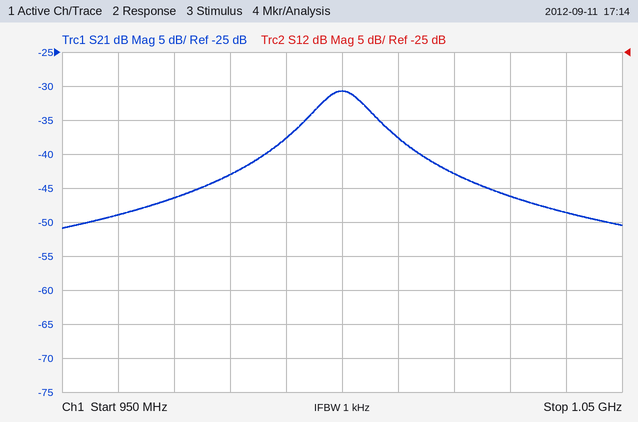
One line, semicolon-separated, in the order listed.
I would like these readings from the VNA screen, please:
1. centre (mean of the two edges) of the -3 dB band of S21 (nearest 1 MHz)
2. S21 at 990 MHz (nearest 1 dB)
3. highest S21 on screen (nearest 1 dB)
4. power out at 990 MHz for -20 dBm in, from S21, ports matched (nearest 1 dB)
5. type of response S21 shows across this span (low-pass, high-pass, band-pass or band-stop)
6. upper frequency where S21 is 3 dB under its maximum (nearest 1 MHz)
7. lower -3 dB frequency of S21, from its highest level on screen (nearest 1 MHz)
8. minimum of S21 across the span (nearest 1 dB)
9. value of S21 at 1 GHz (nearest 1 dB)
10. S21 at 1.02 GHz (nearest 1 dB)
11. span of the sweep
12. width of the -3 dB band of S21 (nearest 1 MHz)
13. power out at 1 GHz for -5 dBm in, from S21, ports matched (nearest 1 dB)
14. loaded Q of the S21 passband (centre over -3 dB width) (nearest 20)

1.000 GHz; -38 dB; -31 dB; -58 dBm; band-pass; 1.005 GHz; 995 MHz; -51 dB; -31 dB; -43 dB; 100 MHz; 10 MHz; -36 dBm; 100
